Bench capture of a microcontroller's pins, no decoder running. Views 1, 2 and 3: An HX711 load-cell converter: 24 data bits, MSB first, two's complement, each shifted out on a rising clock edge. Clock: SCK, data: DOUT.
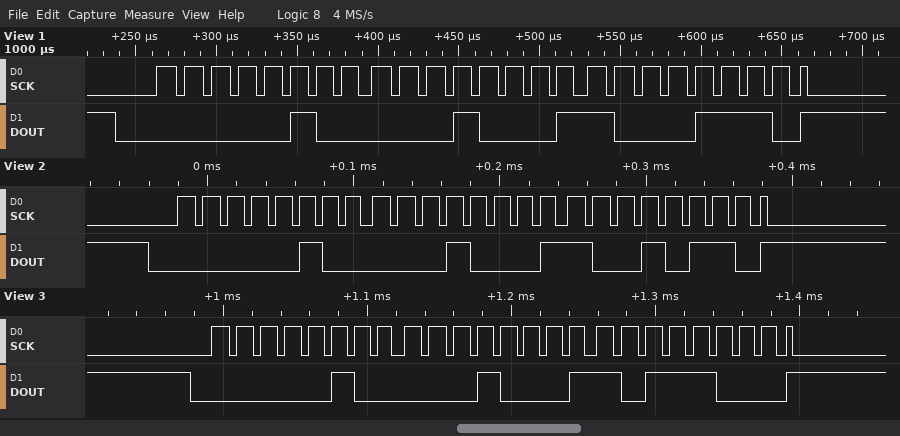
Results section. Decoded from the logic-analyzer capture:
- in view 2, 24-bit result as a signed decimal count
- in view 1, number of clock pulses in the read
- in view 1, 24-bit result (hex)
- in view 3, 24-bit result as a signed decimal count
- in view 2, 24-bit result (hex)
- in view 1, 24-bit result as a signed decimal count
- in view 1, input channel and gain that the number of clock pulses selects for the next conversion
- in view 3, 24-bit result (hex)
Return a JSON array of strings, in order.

["266646", "25", "0x04118E", "266680", "0x041196", "266638", "channel A, gain 128", "0x0411B8"]
